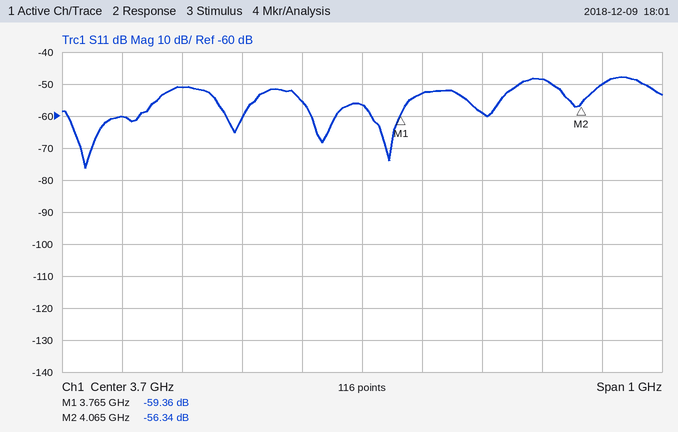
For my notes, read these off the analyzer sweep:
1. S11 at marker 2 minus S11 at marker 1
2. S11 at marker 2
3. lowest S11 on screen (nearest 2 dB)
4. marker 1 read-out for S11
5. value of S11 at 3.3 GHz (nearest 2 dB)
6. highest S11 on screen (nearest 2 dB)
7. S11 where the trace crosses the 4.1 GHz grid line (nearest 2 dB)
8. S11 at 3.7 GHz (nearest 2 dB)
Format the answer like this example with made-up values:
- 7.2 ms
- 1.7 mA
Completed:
- 3.02 dB
- -56.34 dB
- -76 dB
- -59.36 dB
- -60 dB
- -48 dB
- -50 dB
- -56 dB
